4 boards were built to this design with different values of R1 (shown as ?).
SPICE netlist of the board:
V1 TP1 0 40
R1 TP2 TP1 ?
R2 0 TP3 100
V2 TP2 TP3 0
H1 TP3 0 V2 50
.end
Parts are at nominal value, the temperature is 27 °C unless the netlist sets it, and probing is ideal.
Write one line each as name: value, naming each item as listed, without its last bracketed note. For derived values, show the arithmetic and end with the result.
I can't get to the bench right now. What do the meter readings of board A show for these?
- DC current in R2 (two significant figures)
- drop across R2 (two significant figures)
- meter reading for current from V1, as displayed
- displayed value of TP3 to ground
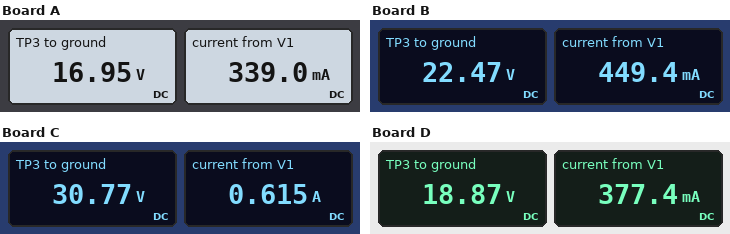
DC current in R2: (16.95 V) / 100 Ω = 170 mA
drop across R2: 16.95 V = 17 V
meter reading for current from V1, as displayed: 339.0 mA
displayed value of TP3 to ground: 16.95 V
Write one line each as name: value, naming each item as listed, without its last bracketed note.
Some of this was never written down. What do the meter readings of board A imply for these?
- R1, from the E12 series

R1, from the E12 series: 68 Ω
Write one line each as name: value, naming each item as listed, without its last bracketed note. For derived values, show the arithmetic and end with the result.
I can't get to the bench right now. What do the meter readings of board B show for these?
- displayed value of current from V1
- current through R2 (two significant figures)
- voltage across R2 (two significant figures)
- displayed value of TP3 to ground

displayed value of current from V1: 449.4 mA
current through R2: (22.47 V) / 100 Ω = 220 mA
voltage across R2: 22.47 V = 22 V
displayed value of TP3 to ground: 22.47 V
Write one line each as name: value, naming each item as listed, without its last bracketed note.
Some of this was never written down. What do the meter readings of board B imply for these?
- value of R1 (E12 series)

value of R1: 39 Ω
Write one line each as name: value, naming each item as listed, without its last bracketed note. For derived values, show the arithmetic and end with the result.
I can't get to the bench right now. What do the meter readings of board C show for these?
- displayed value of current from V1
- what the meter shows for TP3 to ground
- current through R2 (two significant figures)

displayed value of current from V1: 0.615 A
what the meter shows for TP3 to ground: 30.77 V
current through R2: (30.77 V) / 100 Ω = 310 mA
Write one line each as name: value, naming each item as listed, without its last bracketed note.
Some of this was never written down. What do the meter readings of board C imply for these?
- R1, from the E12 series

R1, from the E12 series: 15 Ω
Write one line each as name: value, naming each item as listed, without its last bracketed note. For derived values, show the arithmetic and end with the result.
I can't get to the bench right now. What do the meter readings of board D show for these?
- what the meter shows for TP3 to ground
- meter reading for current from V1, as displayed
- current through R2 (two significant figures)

what the meter shows for TP3 to ground: 18.87 V
meter reading for current from V1, as displayed: 377.4 mA
current through R2: (18.87 V) / 100 Ω = 190 mA
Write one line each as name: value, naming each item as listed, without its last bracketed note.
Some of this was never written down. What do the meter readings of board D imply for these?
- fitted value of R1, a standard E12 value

fitted value of R1, a standard E12 value: 56 Ω
